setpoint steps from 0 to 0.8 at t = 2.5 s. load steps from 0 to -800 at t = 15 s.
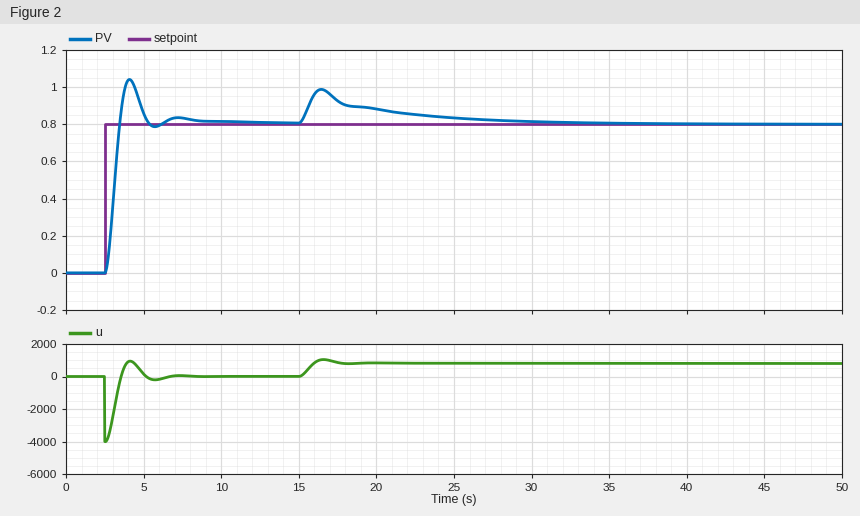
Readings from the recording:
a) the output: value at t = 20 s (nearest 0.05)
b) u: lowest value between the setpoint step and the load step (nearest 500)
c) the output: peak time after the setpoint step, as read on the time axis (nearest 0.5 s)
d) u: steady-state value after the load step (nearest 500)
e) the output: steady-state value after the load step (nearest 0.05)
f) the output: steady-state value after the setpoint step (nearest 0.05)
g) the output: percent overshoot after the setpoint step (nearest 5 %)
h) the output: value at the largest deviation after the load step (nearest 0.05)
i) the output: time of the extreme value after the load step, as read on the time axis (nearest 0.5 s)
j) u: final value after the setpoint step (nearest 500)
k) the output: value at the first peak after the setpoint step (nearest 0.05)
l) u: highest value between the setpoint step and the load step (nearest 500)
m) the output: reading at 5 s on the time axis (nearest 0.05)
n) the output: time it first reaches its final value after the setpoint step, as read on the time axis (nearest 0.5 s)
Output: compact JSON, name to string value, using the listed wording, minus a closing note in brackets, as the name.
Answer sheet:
{"the output: value at t = 20 s": "0.90", "u: lowest value between the setpoint step and the load step": "-4000", "the output: peak time after the setpoint step, as read on the time axis": "4.0 s", "u: steady-state value after the load step": "1000", "the output: steady-state value after the load step": "0.80", "the output: steady-state value after the setpoint step": "0.80", "the output: percent overshoot after the setpoint step": "30 %", "the output: value at the largest deviation after the load step": "1.00", "the output: time of the extreme value after the load step, as read on the time axis": "16.5 s", "u: final value after the setpoint step": "0", "the output: value at the first peak after the setpoint step": "1.05", "u: highest value between the setpoint step and the load step": "1000", "the output: reading at 5 s on the time axis": "0.85", "the output: time it first reaches its final value after the setpoint step, as read on the time axis": "3.5 s"}
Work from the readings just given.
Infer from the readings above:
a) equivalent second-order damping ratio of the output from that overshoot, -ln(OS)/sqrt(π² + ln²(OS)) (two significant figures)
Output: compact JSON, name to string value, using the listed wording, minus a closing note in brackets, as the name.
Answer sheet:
{"equivalent second-order damping ratio of the output from that overshoot, -ln(OS)/sqrt(π² + ln²(OS))": "0.36"}
